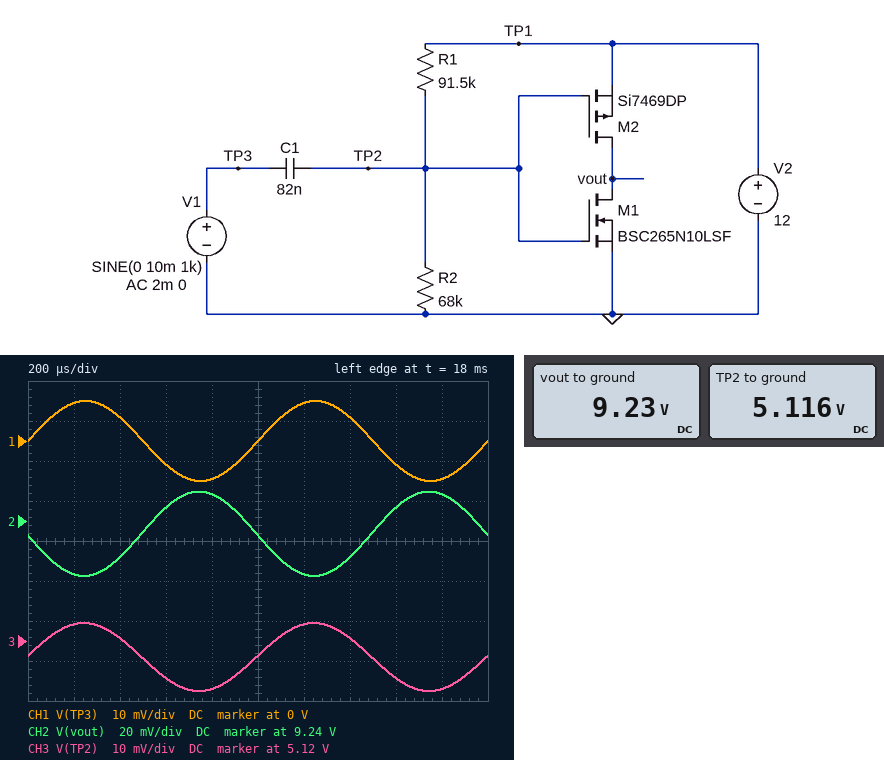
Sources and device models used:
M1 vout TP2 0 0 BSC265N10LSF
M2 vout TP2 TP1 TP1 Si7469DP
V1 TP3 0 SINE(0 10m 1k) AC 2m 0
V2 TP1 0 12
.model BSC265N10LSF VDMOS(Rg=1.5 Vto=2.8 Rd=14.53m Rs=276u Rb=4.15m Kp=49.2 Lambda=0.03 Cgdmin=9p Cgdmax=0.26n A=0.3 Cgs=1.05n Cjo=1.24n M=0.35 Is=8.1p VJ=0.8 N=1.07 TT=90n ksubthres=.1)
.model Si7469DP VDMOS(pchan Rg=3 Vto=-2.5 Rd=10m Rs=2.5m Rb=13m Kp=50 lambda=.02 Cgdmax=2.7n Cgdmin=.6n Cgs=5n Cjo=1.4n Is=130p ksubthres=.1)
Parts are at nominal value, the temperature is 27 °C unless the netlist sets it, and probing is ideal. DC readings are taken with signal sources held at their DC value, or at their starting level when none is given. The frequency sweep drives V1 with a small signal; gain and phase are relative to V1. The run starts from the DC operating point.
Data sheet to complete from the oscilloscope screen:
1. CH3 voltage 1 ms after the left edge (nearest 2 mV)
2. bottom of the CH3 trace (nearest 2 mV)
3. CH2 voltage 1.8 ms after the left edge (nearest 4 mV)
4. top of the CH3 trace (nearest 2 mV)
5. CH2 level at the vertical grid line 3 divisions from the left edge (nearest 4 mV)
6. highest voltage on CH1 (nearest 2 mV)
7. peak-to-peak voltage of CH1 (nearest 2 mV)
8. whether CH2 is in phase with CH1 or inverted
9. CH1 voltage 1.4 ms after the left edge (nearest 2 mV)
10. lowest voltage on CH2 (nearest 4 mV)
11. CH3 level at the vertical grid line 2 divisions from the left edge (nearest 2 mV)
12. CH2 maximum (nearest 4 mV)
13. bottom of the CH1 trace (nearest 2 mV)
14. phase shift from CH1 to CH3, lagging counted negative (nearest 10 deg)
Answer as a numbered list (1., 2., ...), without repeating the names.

1. 5.116 V
2. 5.108 V
3. 9.252 V
4. 5.124 V
5. 9.248 V
6. 10 mV
7. 20 mV
8. inverted
9. 6 mV
10. 9.212 V
11. 5.120 V
12. 9.256 V
13. -10 mV
14. 0 deg
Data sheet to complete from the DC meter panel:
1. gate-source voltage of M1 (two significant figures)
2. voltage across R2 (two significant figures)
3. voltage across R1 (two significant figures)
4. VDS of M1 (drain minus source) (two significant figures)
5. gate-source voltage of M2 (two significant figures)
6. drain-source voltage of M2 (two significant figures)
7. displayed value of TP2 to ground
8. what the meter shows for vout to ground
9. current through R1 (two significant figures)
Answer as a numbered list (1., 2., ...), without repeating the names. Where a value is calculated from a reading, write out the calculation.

1. 5.116 V = 5.1 V
2. 5.116 V = 5.1 V
3. 12 V - 5.116 V = 6.9 V
4. 9.23 V = 9.2 V
5. 5.116 V - 12 V = -6.9 V
6. 9.23 V - 12 V = -2.8 V
7. 5.116 V
8. 9.23 V
9. (12 V - 5.116 V) / 91.5 kΩ = 75 µA
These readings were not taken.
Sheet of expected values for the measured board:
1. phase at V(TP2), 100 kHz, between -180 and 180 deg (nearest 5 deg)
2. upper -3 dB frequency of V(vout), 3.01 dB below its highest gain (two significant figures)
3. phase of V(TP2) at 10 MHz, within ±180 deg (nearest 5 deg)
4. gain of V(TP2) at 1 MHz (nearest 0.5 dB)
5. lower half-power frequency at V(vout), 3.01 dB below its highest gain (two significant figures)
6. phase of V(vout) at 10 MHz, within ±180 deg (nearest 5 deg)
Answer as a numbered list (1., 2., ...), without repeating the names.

1. 0 deg
2. 68 MHz
3. 5 deg
4. -1.5 dB
5. 42 Hz
6. 170 deg
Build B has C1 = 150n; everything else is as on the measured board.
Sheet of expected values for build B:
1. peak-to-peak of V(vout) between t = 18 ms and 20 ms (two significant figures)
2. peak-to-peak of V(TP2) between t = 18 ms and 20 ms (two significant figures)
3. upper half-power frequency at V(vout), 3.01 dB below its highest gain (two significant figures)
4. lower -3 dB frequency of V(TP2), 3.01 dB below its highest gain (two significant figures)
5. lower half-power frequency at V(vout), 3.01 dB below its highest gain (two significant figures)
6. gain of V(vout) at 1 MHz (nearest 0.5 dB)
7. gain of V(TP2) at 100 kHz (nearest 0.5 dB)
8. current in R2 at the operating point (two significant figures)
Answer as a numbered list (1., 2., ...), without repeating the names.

1. 45 mV
2. 18 mV
3. 59 MHz
4. 30 Hz
5. 25 Hz
6. 7.0 dB
7. -1.0 dB
8. 75 µA
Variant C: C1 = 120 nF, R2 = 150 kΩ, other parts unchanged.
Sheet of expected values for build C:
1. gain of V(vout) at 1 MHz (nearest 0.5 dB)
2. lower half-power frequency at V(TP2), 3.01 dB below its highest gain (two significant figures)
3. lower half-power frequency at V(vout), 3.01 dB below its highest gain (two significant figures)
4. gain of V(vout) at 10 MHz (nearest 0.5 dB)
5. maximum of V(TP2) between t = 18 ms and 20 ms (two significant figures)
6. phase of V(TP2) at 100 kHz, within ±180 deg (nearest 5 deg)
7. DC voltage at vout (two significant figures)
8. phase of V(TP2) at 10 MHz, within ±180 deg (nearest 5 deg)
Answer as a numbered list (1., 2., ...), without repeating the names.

1. 4.0 dB
2. 25 Hz
3. 22 Hz
4. 0 dB
5. 7.5 V
6. 0 deg
7. 1.9 V
8. 0 deg
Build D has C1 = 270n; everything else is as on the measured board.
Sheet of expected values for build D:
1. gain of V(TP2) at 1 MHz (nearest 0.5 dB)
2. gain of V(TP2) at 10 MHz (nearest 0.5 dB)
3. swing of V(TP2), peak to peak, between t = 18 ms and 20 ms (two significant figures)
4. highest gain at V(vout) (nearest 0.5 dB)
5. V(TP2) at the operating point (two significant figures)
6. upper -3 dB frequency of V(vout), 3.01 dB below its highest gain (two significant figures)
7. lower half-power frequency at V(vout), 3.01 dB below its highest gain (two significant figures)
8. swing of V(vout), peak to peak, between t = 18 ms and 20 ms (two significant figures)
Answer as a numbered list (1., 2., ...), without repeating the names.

1. -0.5 dB
2. 0 dB
3. 19 mV
4. 7.5 dB
5. 5.1 V
6. 54 MHz
7. 14 Hz
8. 47 mV
